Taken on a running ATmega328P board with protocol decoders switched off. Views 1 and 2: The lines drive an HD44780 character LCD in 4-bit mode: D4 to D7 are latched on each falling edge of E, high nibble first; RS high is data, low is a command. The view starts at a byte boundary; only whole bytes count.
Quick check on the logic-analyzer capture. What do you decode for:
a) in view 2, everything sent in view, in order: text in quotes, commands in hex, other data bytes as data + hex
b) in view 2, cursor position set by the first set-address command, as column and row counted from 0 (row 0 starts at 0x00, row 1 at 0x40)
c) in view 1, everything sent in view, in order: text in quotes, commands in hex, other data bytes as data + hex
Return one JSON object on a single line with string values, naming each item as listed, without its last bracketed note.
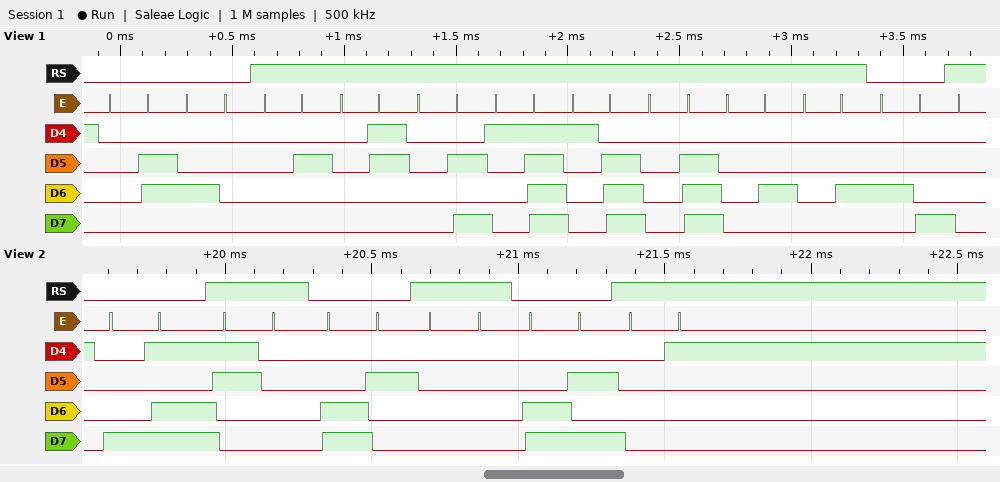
{"in view 2, everything sent in view, in order: text in quotes, commands in hex, other data bytes as data + hex": "0x8D \"0\" 0xC2 data 00 0xCA data 01", "in view 2, cursor position set by the first set-address command, as column and row counted from 0": "column 13, row 0", "in view 1, everything sent in view, in order: text in quotes, commands in hex, other data bytes as data + hex": "0x06 0x40 data 02 03 0A 1F 1E 0E 04 04 0x48"}
